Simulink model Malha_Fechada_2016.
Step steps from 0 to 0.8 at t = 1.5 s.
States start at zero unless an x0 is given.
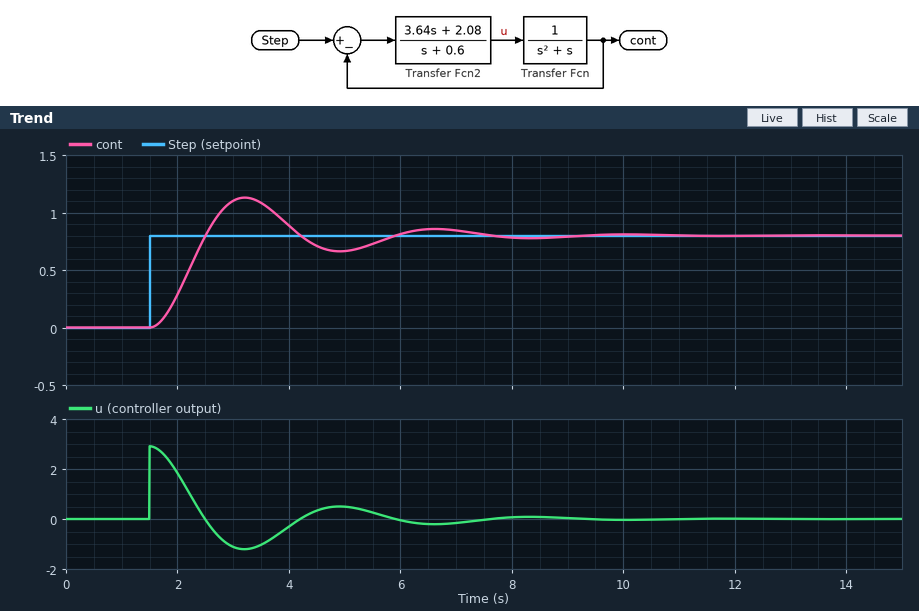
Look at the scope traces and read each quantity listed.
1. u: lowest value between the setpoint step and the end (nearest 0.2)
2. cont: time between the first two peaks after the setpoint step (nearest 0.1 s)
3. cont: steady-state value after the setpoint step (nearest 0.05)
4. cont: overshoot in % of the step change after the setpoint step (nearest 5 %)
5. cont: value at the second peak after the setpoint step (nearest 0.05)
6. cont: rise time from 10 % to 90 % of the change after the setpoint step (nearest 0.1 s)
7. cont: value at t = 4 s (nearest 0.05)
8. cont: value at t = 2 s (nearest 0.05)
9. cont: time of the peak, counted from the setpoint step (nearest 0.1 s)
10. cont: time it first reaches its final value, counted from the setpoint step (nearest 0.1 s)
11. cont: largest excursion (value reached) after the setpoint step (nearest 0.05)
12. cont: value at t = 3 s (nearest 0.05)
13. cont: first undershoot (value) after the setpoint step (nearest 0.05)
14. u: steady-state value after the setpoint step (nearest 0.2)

-1.2
3.4 s
0.80
40 %
0.85
0.7 s
0.90
0.30
1.7 s
1.0 s
1.15
1.10
0.65
0.0
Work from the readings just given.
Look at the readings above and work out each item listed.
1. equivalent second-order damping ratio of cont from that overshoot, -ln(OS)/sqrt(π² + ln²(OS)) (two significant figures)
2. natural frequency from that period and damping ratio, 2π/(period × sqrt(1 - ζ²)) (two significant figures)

0.28
1.9 rad/s
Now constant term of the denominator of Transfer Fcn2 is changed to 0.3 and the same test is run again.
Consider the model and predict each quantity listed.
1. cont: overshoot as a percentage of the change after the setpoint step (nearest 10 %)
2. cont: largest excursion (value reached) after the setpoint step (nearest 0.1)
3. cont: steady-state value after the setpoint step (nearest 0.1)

60 %
1.3
0.8
